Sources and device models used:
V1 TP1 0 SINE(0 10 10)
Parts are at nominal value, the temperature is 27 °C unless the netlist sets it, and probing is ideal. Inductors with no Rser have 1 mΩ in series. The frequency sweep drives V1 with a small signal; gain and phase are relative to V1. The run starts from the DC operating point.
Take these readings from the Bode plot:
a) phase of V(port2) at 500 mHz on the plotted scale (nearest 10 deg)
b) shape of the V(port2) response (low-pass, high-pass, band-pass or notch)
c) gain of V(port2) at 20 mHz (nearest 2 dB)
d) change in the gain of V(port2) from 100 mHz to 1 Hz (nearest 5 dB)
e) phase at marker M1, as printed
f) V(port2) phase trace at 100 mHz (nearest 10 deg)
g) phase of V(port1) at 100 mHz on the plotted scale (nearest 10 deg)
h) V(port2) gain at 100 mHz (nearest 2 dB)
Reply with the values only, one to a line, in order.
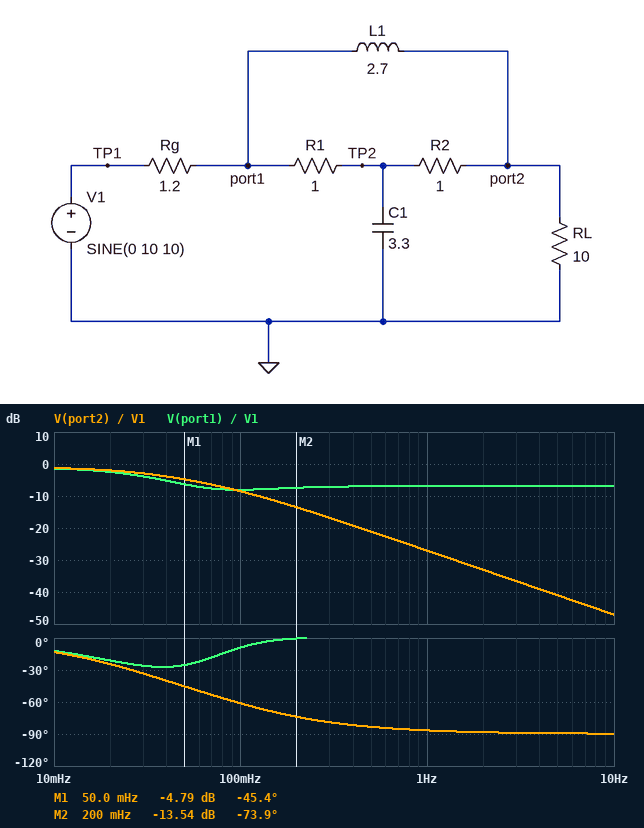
-80 deg
low-pass
-2 dB
-20 dB
-45.4 deg
-60 deg
-10 deg
-8 dB
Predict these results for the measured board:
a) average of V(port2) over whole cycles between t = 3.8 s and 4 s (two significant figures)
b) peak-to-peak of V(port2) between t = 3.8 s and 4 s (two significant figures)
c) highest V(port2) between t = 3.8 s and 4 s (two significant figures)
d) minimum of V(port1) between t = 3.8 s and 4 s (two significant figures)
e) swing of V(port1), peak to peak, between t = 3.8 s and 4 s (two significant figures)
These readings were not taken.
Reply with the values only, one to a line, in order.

12 mV
89 mV
57 mV
-4.5 V
9.1 V
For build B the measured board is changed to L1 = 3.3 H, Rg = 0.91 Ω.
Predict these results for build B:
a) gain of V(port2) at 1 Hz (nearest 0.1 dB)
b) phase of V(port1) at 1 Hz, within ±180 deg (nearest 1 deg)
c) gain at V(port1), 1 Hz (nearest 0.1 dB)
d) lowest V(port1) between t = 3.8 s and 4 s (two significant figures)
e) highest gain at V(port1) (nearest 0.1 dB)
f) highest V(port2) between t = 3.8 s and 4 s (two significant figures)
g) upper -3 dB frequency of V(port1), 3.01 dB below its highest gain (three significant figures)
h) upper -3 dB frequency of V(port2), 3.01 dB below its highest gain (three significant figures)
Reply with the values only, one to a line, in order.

-26.8 dB
0 deg
-5.6 dB
-5.2 V
-0.8 dB
60 mV
36.5 mHz
52.0 mHz
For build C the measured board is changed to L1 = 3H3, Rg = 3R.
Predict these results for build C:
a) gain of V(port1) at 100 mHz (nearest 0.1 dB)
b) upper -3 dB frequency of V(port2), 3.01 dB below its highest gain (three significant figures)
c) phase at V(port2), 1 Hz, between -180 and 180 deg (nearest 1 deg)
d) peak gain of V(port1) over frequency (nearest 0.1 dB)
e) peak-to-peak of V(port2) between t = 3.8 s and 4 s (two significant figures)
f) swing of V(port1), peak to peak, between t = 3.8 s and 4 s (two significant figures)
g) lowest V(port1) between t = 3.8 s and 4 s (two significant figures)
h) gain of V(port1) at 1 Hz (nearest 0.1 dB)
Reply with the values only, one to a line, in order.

-13.3 dB
18.9 mHz
-87 deg
-2.3 dB
44 mV
5.0 V
-2.5 V
-12.1 dB
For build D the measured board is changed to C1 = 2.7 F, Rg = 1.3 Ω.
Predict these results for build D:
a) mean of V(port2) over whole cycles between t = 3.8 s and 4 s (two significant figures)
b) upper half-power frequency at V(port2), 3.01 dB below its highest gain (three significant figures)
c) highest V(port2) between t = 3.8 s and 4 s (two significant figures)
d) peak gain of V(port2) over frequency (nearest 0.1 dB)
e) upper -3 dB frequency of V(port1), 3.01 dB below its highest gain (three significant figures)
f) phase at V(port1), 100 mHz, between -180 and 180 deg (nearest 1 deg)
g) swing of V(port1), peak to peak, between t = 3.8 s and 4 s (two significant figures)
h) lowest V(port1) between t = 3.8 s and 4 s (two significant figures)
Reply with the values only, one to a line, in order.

12 mV
47.0 mHz
59 mV
-1.1 dB
35.3 mHz
-13 deg
8.7 V
-4.3 V
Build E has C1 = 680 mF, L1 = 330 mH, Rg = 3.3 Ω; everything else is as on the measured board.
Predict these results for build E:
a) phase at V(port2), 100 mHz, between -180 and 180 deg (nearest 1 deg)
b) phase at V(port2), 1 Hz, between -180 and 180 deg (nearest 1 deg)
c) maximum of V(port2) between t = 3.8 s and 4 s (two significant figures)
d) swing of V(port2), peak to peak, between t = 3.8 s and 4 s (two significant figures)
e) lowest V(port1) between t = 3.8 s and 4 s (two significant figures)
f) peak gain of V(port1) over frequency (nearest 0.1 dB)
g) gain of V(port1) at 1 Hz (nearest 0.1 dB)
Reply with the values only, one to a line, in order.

-41 deg
-64 deg
160 mV
300 mV
-2.3 V
-2.5 dB
-14.4 dB
